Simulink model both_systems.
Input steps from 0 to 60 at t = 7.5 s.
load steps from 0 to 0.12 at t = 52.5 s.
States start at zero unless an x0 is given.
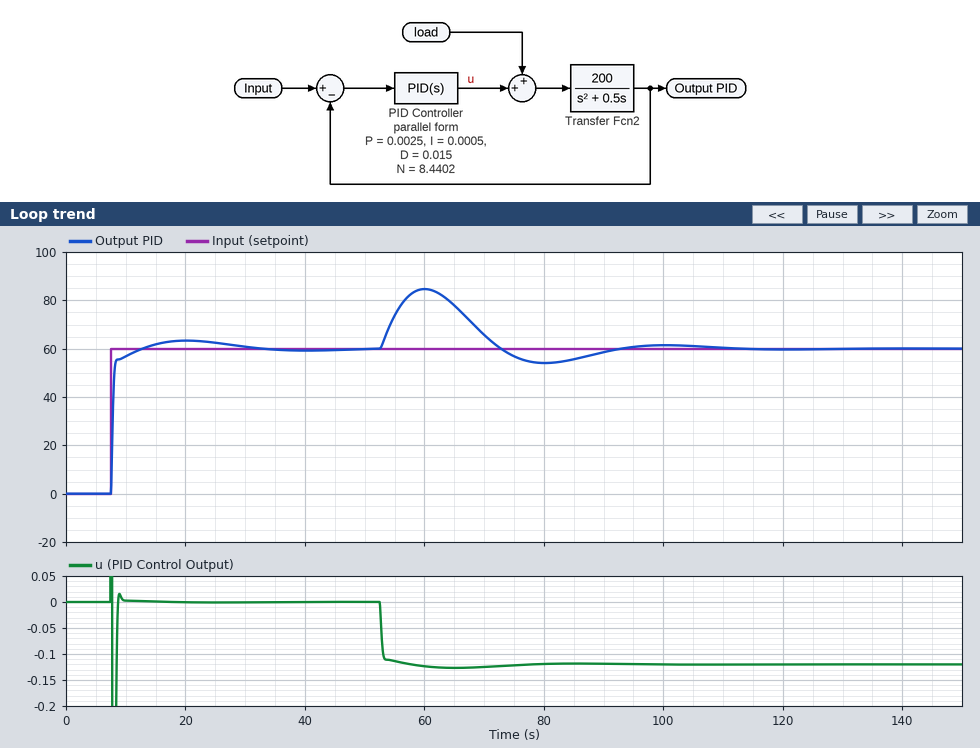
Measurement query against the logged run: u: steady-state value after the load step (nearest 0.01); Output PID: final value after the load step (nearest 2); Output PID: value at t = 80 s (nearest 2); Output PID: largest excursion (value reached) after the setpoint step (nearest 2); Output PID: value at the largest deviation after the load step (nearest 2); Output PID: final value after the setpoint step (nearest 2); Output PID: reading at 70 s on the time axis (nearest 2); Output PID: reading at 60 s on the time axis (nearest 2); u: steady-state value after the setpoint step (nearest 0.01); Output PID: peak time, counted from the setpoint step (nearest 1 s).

-0.12
60
54
64
84
60
66
84
0.00
13 s
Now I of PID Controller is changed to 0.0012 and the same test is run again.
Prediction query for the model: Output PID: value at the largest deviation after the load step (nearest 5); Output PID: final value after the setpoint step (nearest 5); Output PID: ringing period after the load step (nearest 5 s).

80
60
25 s
